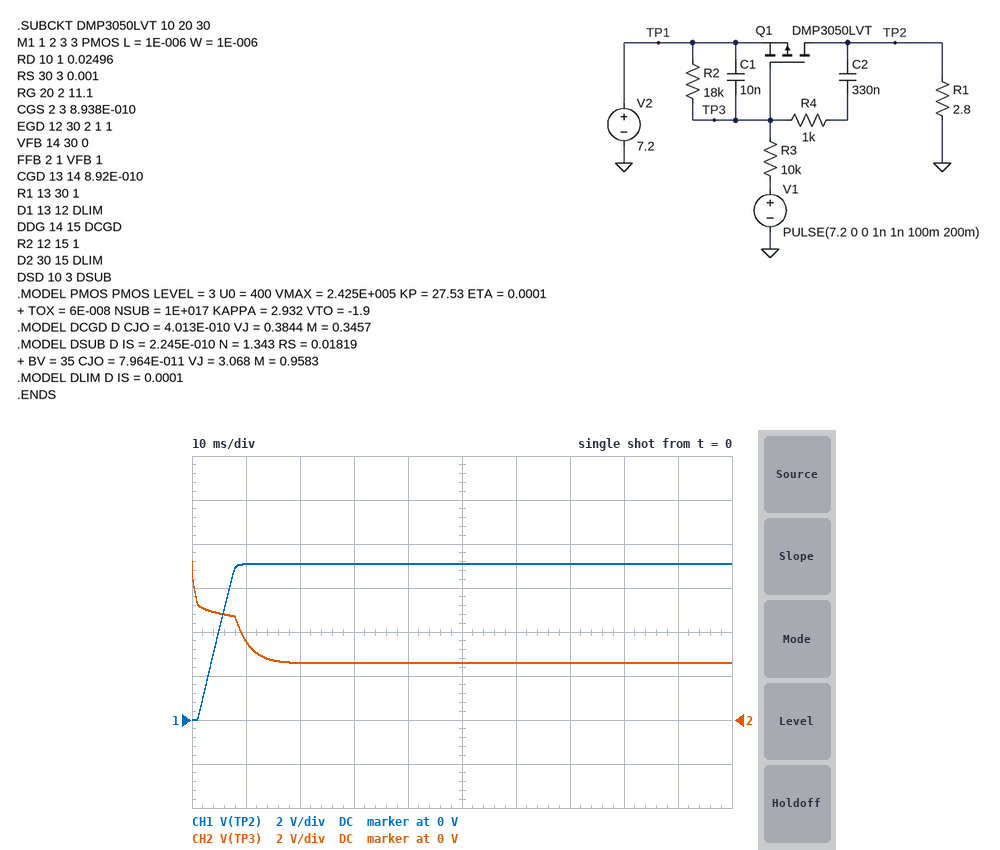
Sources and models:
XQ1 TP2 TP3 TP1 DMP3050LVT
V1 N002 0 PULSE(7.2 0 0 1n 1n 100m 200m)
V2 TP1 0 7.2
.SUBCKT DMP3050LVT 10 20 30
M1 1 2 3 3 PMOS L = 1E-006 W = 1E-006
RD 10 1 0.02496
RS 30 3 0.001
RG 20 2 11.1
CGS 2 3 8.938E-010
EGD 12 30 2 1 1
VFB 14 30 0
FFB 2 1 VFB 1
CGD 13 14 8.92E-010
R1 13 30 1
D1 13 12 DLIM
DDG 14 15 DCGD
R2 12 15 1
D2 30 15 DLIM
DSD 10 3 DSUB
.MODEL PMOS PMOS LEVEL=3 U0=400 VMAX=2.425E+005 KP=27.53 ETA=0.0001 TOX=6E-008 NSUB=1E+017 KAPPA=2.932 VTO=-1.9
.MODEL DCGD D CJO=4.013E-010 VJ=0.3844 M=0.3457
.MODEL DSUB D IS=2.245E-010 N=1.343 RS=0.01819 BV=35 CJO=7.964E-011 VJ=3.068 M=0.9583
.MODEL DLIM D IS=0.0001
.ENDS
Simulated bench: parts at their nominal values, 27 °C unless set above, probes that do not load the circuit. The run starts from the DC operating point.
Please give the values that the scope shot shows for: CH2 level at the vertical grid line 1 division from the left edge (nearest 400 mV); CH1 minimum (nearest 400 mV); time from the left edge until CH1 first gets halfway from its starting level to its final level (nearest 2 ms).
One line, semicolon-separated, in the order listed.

3.6 V; 0 V; 4 ms
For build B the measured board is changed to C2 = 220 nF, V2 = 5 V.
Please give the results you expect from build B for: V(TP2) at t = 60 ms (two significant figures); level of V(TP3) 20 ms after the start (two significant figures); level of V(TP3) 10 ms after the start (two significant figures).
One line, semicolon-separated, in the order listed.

4.9 V; 1.8 V; 2.5 V
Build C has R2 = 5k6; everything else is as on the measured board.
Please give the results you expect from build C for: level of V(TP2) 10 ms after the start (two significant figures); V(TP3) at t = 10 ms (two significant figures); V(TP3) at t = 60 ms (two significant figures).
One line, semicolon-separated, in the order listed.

2.6 V; 4.9 V; 4.6 V
